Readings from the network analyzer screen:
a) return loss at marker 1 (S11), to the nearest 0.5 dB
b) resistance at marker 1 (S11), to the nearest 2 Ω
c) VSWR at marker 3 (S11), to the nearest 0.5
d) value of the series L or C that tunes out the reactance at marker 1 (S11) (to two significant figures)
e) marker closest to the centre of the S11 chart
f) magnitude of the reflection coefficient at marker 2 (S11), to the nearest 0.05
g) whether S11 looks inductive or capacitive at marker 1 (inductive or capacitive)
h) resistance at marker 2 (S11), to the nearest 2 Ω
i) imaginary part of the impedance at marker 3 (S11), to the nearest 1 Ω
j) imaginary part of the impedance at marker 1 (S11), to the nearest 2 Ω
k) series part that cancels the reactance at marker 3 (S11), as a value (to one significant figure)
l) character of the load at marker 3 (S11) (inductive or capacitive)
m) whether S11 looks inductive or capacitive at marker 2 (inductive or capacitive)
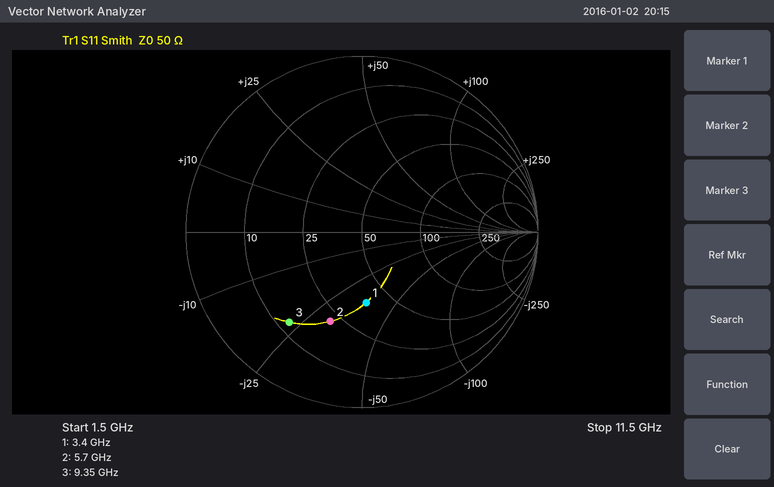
8.0 dB
38 Ω
5.0
1.7 nH
marker 1
0.55
capacitive
22 Ω
-23 Ω
-36 Ω
400 pH
capacitive
capacitive
